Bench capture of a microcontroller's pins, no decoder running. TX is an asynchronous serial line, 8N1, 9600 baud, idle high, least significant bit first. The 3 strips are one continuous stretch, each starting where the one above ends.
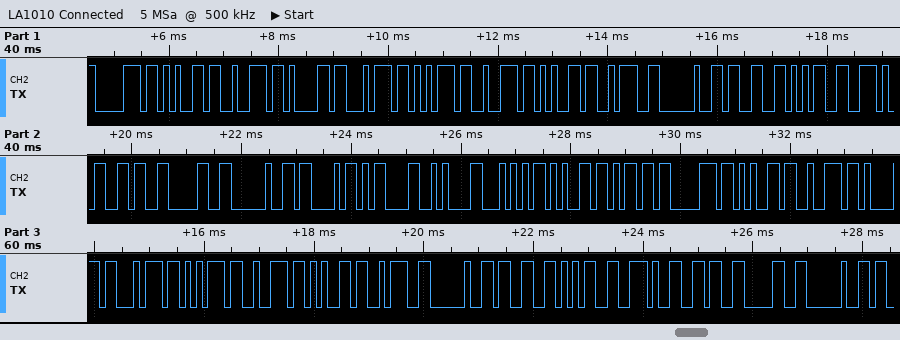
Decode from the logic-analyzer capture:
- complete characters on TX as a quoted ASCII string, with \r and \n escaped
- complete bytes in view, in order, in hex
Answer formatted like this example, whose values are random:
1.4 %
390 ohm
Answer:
"perature: 35.60 C\r\nTemperature: 35.60 "
70 65 72 61 74 75 72 65 3A 20 33 35 2E 36 30 20 43 0D 0A 54 65 6D 70 65 72 61 74 75 72 65 3A 20 33 35 2E 36 30 20
